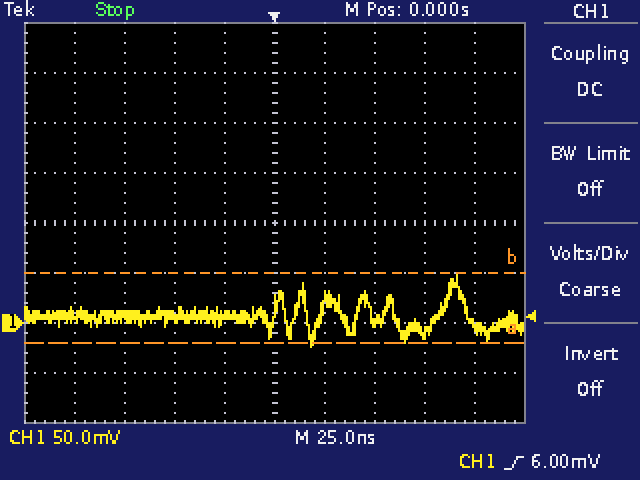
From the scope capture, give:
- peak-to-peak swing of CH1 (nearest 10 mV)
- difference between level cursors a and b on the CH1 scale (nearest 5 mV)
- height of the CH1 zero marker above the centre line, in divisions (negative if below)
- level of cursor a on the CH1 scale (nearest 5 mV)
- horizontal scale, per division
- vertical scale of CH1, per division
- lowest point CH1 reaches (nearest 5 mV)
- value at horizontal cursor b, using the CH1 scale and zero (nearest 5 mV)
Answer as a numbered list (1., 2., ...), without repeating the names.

1. 70 mV
2. 70 mV
3. -2.0 div
4. -20 mV
5. 25 ns
6. 50 mV
7. -25 mV
8. 50 mV
